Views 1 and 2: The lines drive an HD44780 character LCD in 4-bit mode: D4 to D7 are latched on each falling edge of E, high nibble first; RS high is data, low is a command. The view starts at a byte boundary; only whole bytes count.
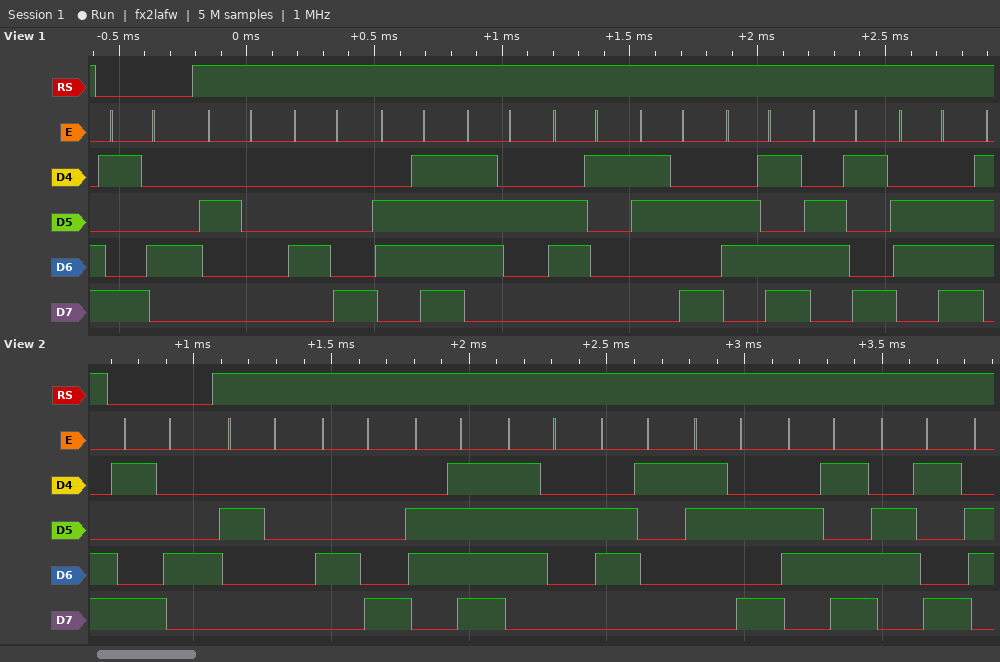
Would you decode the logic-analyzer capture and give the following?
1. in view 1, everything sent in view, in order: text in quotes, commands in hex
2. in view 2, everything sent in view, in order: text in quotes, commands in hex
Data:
0x94 " Hora:min"
0x94 " Hora:mi"
